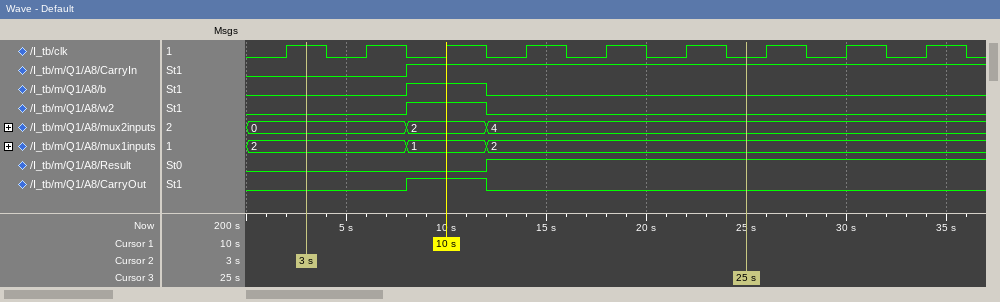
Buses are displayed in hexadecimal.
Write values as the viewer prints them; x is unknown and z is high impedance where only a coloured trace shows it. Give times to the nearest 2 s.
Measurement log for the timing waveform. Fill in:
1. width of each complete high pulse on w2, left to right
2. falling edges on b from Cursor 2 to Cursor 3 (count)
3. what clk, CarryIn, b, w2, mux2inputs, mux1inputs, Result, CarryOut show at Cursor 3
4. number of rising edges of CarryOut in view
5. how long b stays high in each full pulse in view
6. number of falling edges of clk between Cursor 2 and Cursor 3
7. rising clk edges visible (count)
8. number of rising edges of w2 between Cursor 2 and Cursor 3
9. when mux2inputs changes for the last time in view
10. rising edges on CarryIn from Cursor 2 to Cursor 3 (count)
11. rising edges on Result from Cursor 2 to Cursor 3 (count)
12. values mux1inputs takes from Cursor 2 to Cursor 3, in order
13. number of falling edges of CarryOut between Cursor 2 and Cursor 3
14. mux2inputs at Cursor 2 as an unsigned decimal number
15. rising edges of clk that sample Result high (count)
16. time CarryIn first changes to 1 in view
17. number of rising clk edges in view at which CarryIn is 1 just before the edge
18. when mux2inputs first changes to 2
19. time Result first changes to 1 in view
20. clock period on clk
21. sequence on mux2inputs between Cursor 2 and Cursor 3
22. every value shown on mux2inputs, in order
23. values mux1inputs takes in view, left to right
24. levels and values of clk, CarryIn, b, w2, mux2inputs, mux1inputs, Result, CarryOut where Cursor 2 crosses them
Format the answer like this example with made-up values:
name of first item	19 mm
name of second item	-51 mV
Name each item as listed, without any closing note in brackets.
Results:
width of each complete high pulse on w2, left to right	4 s
falling edges on b from Cursor 2 to Cursor 3	1
what clk, CarryIn, b, w2, mux2inputs, mux1inputs, Result, CarryOut show at Cursor 3	clk=0, CarryIn=1, b=0, w2=0, mux2inputs=4, mux1inputs=2, Result=1, CarryOut=0
number of rising edges of CarryOut in view	1
how long b stays high in each full pulse in view	4 s
number of falling edges of clk between Cursor 2 and Cursor 3	6
rising clk edges visible	9
number of rising edges of w2 between Cursor 2 and Cursor 3	1
when mux2inputs changes for the last time in view	12 s
rising edges on CarryIn from Cursor 2 to Cursor 3	1
rising edges on Result from Cursor 2 to Cursor 3	1
values mux1inputs takes from Cursor 2 to Cursor 3, in order	2, 1, 2
number of falling edges of CarryOut between Cursor 2 and Cursor 3	1
mux2inputs at Cursor 2 as an unsigned decimal number	0
rising edges of clk that sample Result high	6
time CarryIn first changes to 1 in view	8 s
number of rising clk edges in view at which CarryIn is 1 just before the edge	7
when mux2inputs first changes to 2	8 s
time Result first changes to 1 in view	12 s
clock period on clk	4 s
sequence on mux2inputs between Cursor 2 and Cursor 3	0, 2, 4
every value shown on mux2inputs, in order	0, 2, 4
values mux1inputs takes in view, left to right	2, 1, 2
levels and values of clk, CarryIn, b, w2, mux2inputs, mux1inputs, Result, CarryOut where Cursor 2 crosses them	clk=1, CarryIn=0, b=0, w2=0, mux2inputs=0, mux1inputs=2, Result=0, CarryOut=0
